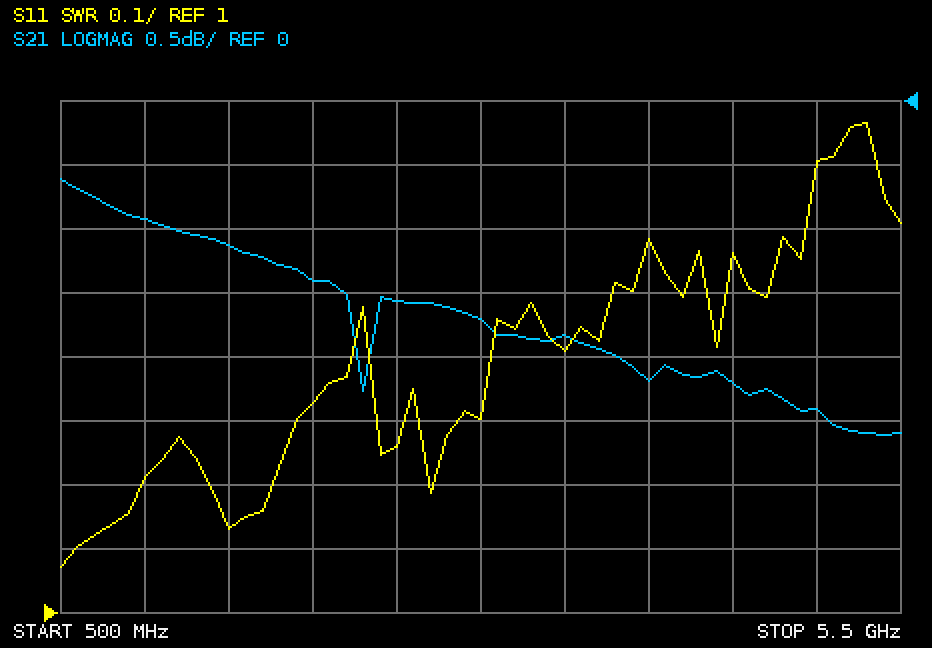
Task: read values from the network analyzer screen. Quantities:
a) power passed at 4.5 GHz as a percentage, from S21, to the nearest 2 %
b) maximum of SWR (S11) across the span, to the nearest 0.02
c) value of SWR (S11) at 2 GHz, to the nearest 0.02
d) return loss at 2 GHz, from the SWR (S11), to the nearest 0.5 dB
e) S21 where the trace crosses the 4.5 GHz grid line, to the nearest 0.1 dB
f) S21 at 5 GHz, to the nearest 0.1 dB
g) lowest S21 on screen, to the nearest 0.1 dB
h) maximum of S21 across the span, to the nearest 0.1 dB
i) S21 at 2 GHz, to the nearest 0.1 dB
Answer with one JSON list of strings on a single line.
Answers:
["60 %", "1.76", "1.32", "17.0 dB", "-2.2 dB", "-2.4 dB", "-2.6 dB", "-0.6 dB", "-1.4 dB"]
